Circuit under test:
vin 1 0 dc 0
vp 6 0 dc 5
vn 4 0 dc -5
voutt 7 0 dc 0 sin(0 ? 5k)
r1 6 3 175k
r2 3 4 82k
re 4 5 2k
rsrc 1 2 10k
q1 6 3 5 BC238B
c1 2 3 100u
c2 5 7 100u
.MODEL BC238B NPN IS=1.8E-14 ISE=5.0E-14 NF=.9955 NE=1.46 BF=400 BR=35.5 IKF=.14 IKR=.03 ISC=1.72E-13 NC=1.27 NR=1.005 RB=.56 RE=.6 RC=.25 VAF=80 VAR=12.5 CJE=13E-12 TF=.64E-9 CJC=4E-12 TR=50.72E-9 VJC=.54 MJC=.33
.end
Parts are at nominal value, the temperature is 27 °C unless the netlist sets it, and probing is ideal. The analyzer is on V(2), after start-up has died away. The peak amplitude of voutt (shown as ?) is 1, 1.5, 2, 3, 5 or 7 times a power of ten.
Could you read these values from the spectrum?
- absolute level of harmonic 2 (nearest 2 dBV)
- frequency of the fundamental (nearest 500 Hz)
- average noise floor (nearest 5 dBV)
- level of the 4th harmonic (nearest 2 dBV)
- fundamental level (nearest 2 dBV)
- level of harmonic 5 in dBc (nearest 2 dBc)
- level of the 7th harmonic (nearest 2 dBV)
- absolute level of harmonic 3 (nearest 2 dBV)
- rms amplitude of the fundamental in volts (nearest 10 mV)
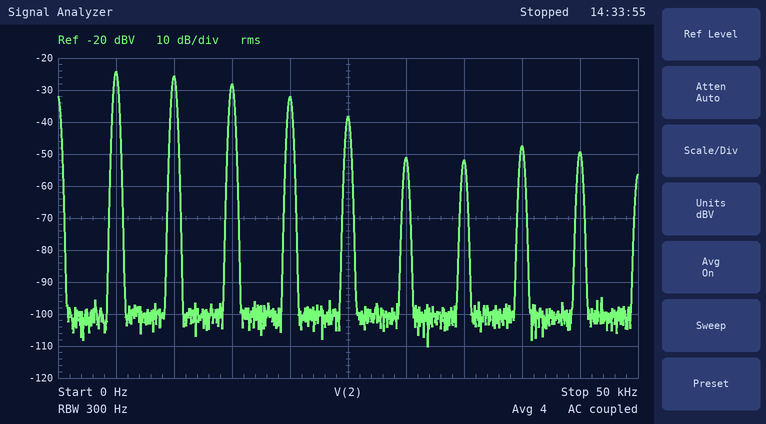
-26 dBV
5.0 kHz
-100 dBV
-32 dBV
-24 dBV
-14 dBc
-52 dBV
-28 dBV
60 mV
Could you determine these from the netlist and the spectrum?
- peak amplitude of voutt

1.5 V
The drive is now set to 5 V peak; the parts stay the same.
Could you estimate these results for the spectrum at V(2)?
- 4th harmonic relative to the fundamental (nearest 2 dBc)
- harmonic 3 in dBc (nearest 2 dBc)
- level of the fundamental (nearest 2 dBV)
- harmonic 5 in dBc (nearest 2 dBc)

-4 dBc
-2 dBc
-18 dBV
-8 dBc
